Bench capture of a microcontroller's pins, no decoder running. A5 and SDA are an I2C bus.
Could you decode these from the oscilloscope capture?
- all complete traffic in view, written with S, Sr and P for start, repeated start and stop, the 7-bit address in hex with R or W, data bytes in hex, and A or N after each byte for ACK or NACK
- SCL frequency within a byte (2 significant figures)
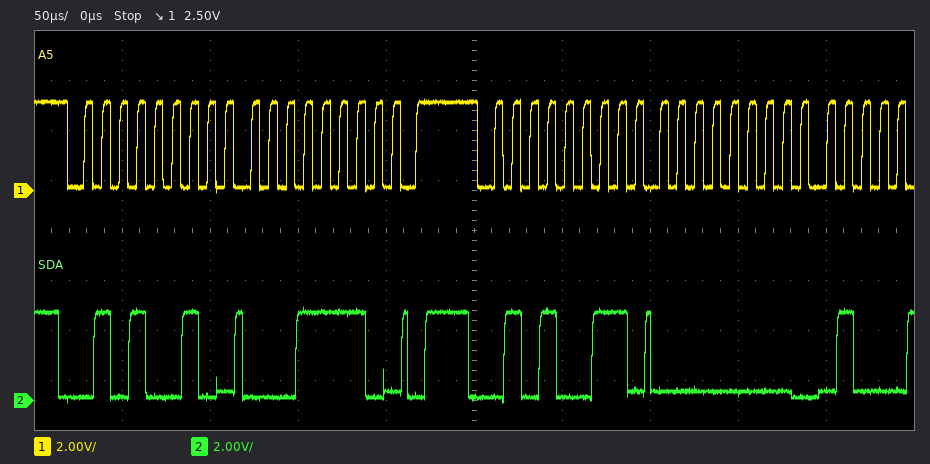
S 29W A 1E A P S 29R A 00 A
100 kHz
